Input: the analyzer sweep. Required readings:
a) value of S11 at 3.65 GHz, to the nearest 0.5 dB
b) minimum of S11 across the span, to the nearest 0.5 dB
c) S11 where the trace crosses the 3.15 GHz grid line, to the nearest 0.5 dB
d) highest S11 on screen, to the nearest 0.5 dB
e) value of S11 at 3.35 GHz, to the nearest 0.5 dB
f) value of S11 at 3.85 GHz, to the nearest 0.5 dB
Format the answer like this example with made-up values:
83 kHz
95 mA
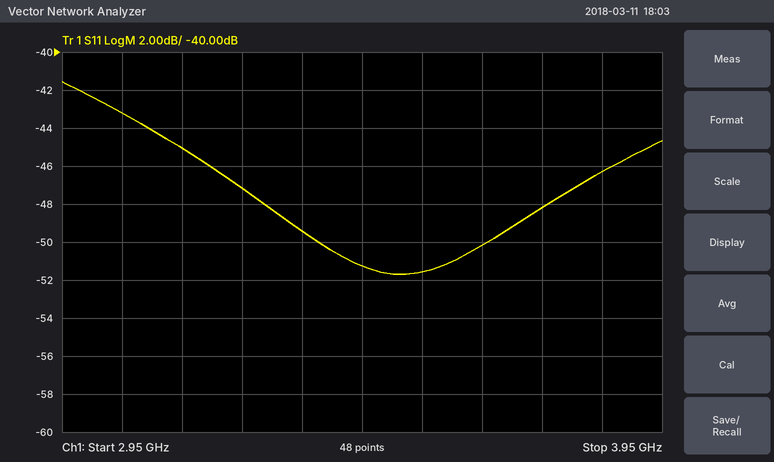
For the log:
-50.0 dB
-51.5 dB
-45.0 dB
-41.5 dB
-49.5 dB
-46.5 dB
